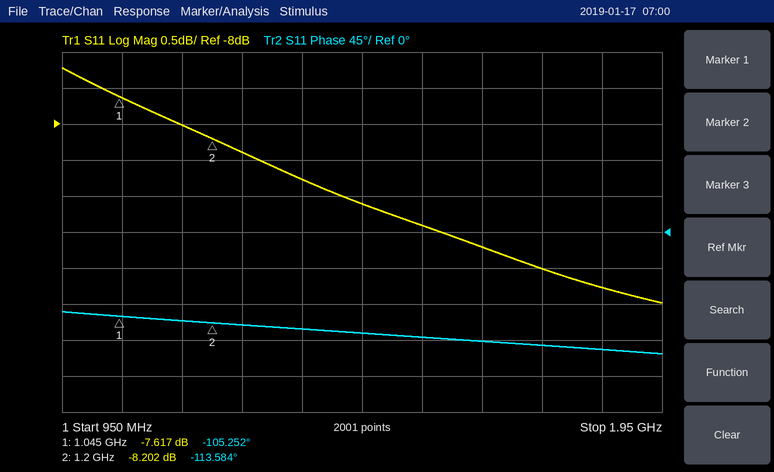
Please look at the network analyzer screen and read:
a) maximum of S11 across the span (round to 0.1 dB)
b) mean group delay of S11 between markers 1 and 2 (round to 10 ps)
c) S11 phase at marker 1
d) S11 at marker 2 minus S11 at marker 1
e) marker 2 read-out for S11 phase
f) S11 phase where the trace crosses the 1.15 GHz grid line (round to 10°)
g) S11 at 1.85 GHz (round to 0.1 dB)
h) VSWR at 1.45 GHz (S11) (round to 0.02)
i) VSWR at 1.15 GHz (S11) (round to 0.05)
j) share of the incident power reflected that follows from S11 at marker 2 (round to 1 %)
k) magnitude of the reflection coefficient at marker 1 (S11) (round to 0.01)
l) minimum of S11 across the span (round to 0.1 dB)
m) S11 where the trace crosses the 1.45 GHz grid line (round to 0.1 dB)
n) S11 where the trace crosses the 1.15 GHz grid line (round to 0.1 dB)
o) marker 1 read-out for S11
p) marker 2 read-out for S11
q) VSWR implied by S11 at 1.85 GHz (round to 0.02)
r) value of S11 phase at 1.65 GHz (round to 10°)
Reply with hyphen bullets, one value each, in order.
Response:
- -7.2 dB
- 150 ps
- -105.252°
- -0.585 dB
- -113.584°
- -110°
- -10.3 dB
- 2.08
- 2.30
- 15 %
- 0.42
- -10.5 dB
- -9.1 dB
- -8.0 dB
- -7.617 dB
- -8.202 dB
- 1.88
- -140°
